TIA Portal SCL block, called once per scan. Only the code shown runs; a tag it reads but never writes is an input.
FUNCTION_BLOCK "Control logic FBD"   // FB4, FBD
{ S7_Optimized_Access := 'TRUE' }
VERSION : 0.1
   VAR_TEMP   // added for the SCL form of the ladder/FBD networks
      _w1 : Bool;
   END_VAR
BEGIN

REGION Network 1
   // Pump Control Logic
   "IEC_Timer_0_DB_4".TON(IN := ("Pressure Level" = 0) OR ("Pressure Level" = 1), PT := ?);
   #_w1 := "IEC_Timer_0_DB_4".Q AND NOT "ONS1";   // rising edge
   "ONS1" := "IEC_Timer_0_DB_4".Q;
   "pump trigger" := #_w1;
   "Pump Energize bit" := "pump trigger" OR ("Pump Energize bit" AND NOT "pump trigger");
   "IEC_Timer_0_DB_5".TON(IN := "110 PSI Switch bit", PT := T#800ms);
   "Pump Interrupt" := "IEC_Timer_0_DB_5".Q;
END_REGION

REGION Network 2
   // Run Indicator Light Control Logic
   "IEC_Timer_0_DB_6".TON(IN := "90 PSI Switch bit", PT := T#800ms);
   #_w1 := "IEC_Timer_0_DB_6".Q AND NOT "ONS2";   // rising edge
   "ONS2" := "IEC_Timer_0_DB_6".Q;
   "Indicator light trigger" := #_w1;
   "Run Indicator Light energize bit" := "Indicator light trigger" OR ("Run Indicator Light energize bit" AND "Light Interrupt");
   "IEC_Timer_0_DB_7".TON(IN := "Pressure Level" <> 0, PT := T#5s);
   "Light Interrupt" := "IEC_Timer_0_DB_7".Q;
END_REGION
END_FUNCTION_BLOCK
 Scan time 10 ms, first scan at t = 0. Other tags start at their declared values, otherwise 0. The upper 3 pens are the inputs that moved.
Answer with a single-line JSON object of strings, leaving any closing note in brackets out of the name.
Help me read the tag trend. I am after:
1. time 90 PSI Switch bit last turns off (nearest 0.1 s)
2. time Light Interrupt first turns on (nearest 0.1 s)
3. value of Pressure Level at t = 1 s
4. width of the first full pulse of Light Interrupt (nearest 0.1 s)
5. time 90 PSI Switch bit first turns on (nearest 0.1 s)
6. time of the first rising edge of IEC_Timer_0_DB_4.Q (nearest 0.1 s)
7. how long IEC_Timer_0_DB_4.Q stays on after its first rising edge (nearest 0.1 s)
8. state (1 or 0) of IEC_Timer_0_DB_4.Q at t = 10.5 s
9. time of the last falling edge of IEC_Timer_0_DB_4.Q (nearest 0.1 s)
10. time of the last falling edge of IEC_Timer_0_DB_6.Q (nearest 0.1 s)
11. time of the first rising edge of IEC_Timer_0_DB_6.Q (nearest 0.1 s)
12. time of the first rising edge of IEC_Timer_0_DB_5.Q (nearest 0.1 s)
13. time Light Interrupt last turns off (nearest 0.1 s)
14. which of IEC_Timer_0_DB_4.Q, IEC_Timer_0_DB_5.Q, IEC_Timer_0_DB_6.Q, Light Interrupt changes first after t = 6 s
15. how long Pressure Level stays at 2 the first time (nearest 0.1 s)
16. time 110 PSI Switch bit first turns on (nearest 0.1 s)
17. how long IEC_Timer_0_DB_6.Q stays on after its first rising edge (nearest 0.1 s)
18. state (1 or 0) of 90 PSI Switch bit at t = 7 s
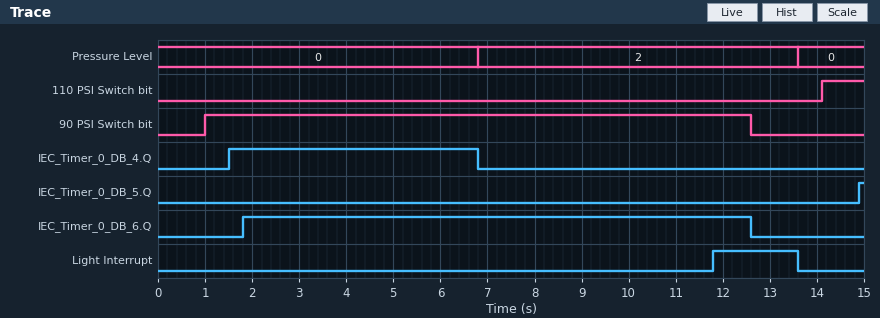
{"time 90 PSI Switch bit last turns off": "12.6 s", "time Light Interrupt first turns on": "11.8 s", "value of Pressure Level at t = 1 s": "0", "width of the first full pulse of Light Interrupt": "1.8 s", "time 90 PSI Switch bit first turns on": "1.0 s", "time of the first rising edge of IEC_Timer_0_DB_4.Q": "1.5 s", "how long IEC_Timer_0_DB_4.Q stays on after its first rising edge": "5.3 s", "state (1 or 0) of IEC_Timer_0_DB_4.Q at t = 10.5 s": "0", "time of the last falling edge of IEC_Timer_0_DB_4.Q": "6.8 s", "time of the last falling edge of IEC_Timer_0_DB_6.Q": "12.6 s", "time of the first rising edge of IEC_Timer_0_DB_6.Q": "1.8 s", "time of the first rising edge of IEC_Timer_0_DB_5.Q": "14.9 s", "time Light Interrupt last turns off": "13.6 s", "which of IEC_Timer_0_DB_4.Q, IEC_Timer_0_DB_5.Q, IEC_Timer_0_DB_6.Q, Light Interrupt changes first after t = 6 s": "IEC_Timer_0_DB_4.Q", "how long Pressure Level stays at 2 the first time": "6.8 s", "time 110 PSI Switch bit first turns on": "14.1 s", "how long IEC_Timer_0_DB_6.Q stays on after its first rising edge": "10.8 s", "state (1 or 0) of 90 PSI Switch bit at t = 7 s": "1"}
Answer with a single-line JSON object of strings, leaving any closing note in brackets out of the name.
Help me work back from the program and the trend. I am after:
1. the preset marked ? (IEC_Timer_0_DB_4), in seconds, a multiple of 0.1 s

{"the preset marked ? (IEC_Timer_0_DB_4), in seconds, a multiple of 0.1 s": "1.5 s"}
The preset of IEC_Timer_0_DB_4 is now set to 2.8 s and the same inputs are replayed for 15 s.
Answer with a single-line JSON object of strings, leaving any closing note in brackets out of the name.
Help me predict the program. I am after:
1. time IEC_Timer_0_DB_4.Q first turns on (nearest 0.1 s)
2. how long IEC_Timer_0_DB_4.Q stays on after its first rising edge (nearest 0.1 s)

{"time IEC_Timer_0_DB_4.Q first turns on": "2.8 s", "how long IEC_Timer_0_DB_4.Q stays on after its first rising edge": "4.0 s"}
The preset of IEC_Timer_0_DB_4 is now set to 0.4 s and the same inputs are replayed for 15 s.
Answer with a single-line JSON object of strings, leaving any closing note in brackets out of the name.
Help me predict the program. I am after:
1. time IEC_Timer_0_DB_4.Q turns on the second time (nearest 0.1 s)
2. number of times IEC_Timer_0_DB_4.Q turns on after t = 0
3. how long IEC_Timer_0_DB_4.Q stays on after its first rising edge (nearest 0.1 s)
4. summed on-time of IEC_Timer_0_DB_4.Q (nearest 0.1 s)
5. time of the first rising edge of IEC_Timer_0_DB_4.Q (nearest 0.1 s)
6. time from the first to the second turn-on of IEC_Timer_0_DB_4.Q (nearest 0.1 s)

{"time IEC_Timer_0_DB_4.Q turns on the second time": "14.0 s", "number of times IEC_Timer_0_DB_4.Q turns on after t = 0": "2", "how long IEC_Timer_0_DB_4.Q stays on after its first rising edge": "6.4 s", "summed on-time of IEC_Timer_0_DB_4.Q": "7.4 s", "time of the first rising edge of IEC_Timer_0_DB_4.Q": "0.4 s", "time from the first to the second turn-on of IEC_Timer_0_DB_4.Q": "13.6 s"}
